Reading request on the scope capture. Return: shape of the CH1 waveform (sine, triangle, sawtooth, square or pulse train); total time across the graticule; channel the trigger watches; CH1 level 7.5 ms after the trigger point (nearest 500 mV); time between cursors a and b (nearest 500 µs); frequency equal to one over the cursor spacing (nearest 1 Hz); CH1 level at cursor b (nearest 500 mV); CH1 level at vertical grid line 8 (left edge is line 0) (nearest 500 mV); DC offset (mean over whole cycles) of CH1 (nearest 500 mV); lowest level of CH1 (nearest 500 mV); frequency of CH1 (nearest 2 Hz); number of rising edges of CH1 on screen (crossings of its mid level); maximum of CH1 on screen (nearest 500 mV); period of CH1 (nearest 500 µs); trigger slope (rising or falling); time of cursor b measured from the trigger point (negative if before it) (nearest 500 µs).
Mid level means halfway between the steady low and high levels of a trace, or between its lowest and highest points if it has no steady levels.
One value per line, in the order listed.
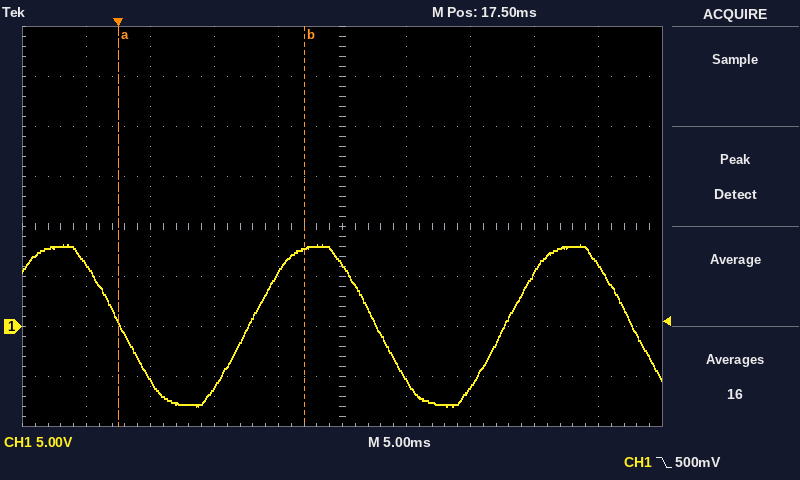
sine
50 ms
CH1
-6.0 V
14.5 ms
69 Hz
8.0 V
5.5 V
0.0 V
-8.0 V
50 Hz
2
8.0 V
20.0 ms
falling
+14.5 ms
